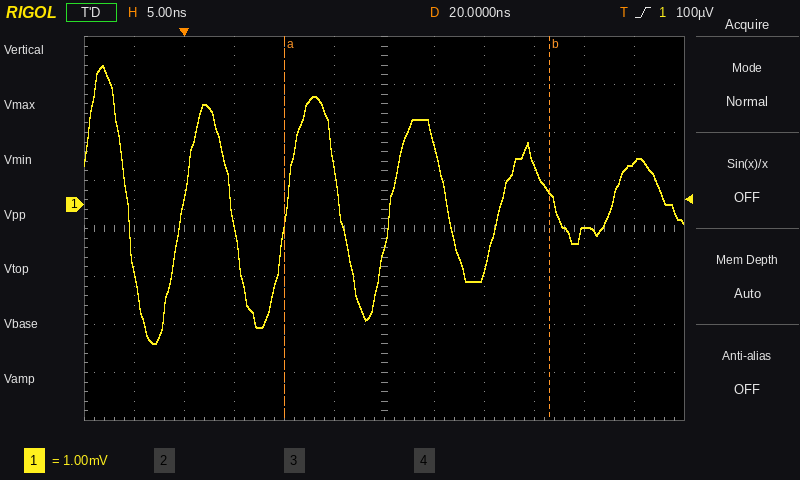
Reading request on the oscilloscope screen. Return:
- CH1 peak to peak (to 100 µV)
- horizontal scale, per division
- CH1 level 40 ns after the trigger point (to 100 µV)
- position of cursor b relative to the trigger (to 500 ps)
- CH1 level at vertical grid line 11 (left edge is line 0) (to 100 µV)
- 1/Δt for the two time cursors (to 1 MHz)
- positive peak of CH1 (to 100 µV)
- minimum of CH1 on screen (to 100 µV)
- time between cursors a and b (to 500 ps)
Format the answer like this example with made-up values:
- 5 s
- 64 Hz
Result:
- 5.8 mV
- 5 ns
- -500 µV
- +36.5 ns
- 900 µV
- 38 MHz
- 2.9 mV
- -2.9 mV
- 26.5 ns
